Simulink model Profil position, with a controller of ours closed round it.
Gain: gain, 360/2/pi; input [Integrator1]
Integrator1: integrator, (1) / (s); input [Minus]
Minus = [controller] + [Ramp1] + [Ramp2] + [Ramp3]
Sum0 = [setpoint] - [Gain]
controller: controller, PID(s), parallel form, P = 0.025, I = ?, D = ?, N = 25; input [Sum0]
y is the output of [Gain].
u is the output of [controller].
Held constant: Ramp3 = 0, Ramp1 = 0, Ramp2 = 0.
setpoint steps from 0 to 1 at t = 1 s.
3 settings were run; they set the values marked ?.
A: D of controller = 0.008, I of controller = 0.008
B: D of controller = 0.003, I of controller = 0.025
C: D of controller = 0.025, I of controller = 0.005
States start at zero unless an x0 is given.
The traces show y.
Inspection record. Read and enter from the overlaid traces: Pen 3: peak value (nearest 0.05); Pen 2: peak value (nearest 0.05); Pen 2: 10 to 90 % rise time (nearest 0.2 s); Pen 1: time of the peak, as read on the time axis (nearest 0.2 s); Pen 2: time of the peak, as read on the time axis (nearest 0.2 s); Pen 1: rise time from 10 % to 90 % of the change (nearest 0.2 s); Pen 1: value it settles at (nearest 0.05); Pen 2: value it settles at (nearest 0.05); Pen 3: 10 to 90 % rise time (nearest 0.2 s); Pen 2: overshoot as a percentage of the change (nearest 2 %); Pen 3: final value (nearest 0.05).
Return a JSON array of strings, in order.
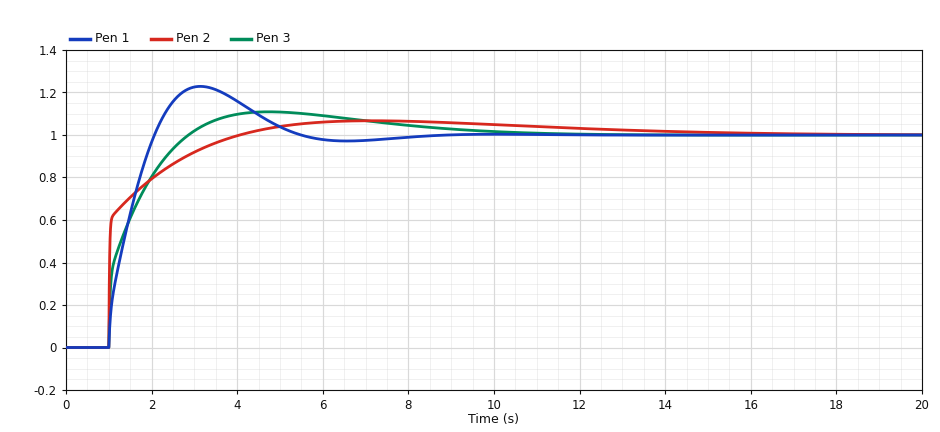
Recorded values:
["1.10", "1.05", "1.8 s", "3.2 s", "7.2 s", "0.8 s", "1.00", "1.00", "1.4 s", "6 %", "1.00"]
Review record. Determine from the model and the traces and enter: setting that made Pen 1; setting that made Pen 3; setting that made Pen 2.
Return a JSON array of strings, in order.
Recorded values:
["B", "A", "C"]
